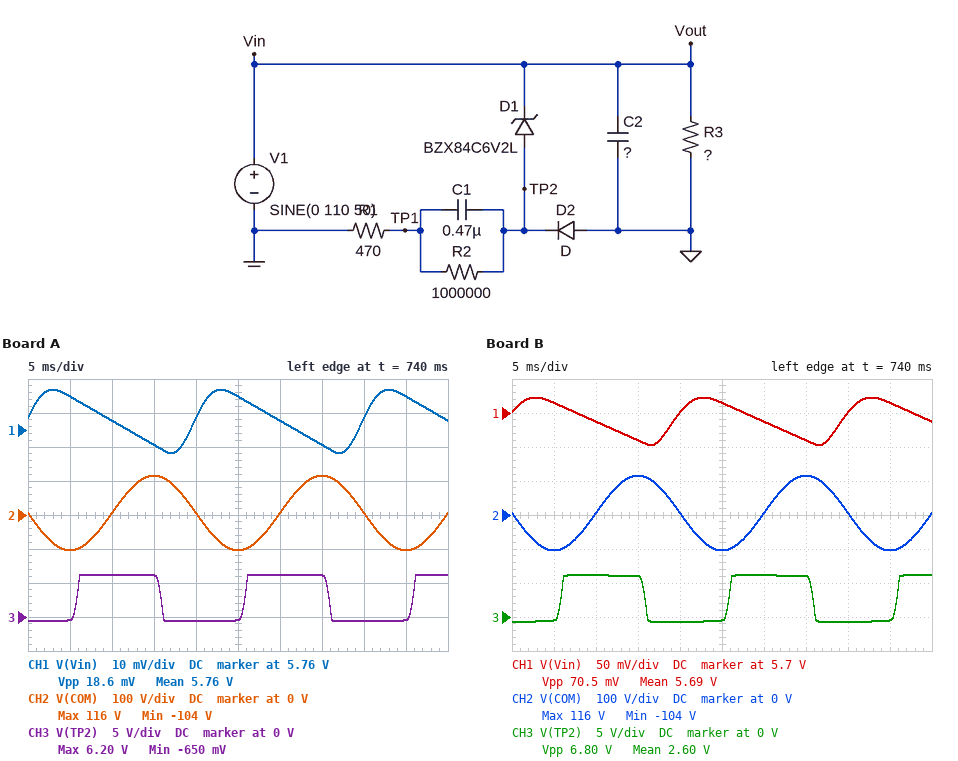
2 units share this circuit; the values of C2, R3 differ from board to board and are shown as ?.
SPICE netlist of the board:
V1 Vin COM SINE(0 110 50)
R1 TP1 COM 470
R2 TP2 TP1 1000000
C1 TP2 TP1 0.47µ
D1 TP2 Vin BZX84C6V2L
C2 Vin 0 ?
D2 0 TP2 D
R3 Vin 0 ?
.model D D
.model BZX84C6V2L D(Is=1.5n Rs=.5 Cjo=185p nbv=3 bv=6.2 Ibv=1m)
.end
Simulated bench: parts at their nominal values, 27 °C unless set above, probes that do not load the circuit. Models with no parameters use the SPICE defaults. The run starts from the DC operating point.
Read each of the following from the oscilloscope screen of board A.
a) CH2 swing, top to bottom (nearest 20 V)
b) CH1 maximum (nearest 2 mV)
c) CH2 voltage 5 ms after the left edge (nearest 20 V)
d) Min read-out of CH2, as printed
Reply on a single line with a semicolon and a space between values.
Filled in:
220 V; 5.772 V; -100 V; -104 V
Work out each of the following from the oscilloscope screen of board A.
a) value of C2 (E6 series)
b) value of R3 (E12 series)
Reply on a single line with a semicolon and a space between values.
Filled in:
150 µF; 27 kΩ
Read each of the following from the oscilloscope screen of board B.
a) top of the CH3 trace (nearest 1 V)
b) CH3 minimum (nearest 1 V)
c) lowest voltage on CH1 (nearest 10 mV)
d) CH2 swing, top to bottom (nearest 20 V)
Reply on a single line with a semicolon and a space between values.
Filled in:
6 V; -1 V; 5.65 V; 220 V
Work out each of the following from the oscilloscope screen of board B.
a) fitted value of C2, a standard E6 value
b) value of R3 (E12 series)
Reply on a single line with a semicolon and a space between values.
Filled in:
220 µF; 4.7 kΩ
